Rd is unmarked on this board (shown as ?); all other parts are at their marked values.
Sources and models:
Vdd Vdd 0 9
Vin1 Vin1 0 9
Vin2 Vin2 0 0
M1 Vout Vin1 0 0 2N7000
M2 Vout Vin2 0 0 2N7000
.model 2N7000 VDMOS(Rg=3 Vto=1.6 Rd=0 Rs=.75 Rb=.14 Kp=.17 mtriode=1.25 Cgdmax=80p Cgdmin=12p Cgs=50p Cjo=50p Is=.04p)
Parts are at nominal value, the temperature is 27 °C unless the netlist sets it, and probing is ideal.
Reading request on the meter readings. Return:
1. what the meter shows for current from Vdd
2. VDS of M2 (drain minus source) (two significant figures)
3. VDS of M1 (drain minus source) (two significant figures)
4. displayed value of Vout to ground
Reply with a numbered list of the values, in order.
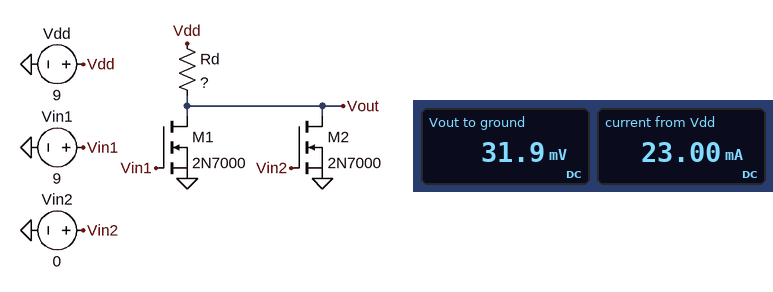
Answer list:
1. 23.00 mA
2. 32 mV
3. 32 mV
4. 31.9 mV
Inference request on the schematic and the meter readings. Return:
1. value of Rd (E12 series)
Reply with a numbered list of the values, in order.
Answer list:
1. 390 Ω
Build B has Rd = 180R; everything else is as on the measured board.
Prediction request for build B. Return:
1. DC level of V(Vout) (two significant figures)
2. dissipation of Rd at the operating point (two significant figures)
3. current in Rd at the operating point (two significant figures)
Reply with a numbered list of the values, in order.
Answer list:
1. 69 mV
2. 440 mW
3. 50 mA
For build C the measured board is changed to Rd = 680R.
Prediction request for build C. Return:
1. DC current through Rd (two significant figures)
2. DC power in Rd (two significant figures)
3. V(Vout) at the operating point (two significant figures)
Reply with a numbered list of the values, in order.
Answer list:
1. 13 mA
2. 120 mW
3. 18 mV
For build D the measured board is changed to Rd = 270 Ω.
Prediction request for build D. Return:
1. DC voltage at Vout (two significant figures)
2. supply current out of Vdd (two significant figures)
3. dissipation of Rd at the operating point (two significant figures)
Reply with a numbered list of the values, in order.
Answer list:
1. 46 mV
2. 33 mA
3. 300 mW
